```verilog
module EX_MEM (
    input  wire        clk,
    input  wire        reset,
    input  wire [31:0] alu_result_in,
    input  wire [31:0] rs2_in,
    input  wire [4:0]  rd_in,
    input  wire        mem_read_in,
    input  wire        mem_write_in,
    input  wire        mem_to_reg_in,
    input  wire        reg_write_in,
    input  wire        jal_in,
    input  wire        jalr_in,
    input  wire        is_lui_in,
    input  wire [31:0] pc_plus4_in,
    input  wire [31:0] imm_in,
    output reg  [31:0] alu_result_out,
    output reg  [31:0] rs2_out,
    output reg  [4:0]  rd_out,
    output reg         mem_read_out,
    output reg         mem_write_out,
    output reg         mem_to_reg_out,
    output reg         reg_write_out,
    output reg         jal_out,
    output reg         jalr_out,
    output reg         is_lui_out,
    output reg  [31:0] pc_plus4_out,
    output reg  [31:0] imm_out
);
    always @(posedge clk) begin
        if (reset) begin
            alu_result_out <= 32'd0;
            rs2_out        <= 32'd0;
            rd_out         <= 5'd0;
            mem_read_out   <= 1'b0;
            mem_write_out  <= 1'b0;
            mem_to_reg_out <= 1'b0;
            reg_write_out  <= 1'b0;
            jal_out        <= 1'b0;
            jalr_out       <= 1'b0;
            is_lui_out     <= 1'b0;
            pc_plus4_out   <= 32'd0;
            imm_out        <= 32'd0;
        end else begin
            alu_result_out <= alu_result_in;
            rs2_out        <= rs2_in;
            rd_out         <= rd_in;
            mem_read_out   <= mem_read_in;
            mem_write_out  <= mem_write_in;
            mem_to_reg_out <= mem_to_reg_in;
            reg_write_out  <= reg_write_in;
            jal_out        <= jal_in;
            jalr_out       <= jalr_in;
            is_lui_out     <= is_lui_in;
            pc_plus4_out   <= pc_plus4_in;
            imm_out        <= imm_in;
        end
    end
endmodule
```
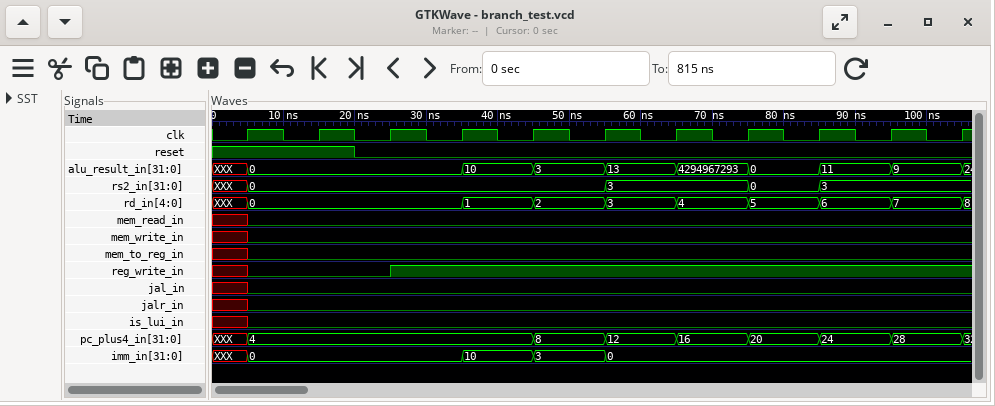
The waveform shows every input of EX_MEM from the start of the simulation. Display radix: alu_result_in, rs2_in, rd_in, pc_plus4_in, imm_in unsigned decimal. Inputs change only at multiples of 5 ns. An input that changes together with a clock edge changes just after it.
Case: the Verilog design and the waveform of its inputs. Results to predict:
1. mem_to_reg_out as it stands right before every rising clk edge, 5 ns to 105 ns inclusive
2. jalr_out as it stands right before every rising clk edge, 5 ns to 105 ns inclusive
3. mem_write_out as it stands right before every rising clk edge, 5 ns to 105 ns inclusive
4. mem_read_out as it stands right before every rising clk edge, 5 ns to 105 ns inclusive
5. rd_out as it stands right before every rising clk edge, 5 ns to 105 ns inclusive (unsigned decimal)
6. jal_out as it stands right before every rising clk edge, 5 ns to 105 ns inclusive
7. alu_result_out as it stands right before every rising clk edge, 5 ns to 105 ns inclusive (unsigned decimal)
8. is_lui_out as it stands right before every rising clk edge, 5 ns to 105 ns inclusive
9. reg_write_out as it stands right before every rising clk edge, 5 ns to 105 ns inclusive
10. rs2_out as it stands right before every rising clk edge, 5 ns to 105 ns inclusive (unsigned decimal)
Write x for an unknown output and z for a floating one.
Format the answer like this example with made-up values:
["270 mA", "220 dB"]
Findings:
["x 0 0 0 0 0 0 0 0 0 0", "x 0 0 0 0 0 0 0 0 0 0", "x 0 0 0 0 0 0 0 0 0 0", "x 0 0 0 0 0 0 0 0 0 0", "x, 0, 0, 0, 0, 1, 2, 3, 4, 5, 6", "x 0 0 0 0 0 0 0 0 0 0", "x, 0, 0, 0, 0, 10, 3, 13, 4294967293, 0, 11", "x 0 0 0 0 0 0 0 0 0 0", "x 0 0 0 1 1 1 1 1 1 1", "x, 0, 0, 0, 0, 0, 0, 3, 3, 0, 3"]
